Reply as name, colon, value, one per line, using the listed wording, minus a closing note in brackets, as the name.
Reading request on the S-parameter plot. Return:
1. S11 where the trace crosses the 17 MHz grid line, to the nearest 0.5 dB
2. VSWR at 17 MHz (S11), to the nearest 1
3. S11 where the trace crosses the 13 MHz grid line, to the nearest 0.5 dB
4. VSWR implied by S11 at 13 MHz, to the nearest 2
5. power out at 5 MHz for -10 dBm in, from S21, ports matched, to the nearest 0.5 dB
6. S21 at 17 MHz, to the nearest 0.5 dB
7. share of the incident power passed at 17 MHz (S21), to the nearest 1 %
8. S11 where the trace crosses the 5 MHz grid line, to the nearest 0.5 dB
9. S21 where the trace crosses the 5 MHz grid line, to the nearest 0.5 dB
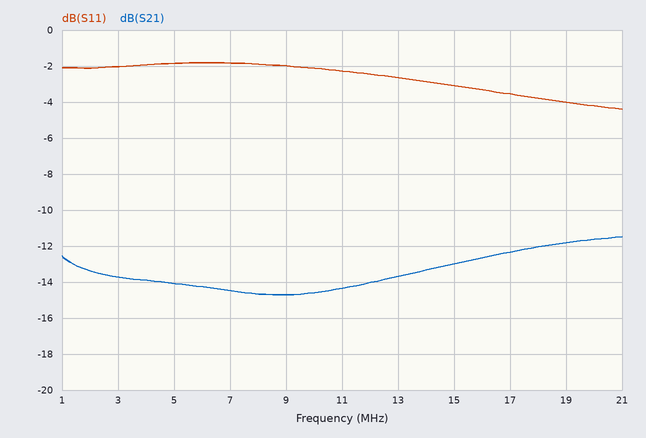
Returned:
S11 where the trace crosses the 17 MHz grid line, to the nearest 0.5 dB: -3.5 dB
VSWR at 17 MHz (S11), to the nearest 1: 5
S11 where the trace crosses the 13 MHz grid line, to the nearest 0.5 dB: -2.5 dB
VSWR implied by S11 at 13 MHz, to the nearest 2: 6
power out at 5 MHz for -10 dBm in, from S21, ports matched, to the nearest 0.5 dB: -24.0 dBm
S21 at 17 MHz, to the nearest 0.5 dB: -12.5 dB
share of the incident power passed at 17 MHz (S21), to the nearest 1 %: 6 %
S11 where the trace crosses the 5 MHz grid line, to the nearest 0.5 dB: -2.0 dB
S21 where the trace crosses the 5 MHz grid line, to the nearest 0.5 dB: -14.0 dB
